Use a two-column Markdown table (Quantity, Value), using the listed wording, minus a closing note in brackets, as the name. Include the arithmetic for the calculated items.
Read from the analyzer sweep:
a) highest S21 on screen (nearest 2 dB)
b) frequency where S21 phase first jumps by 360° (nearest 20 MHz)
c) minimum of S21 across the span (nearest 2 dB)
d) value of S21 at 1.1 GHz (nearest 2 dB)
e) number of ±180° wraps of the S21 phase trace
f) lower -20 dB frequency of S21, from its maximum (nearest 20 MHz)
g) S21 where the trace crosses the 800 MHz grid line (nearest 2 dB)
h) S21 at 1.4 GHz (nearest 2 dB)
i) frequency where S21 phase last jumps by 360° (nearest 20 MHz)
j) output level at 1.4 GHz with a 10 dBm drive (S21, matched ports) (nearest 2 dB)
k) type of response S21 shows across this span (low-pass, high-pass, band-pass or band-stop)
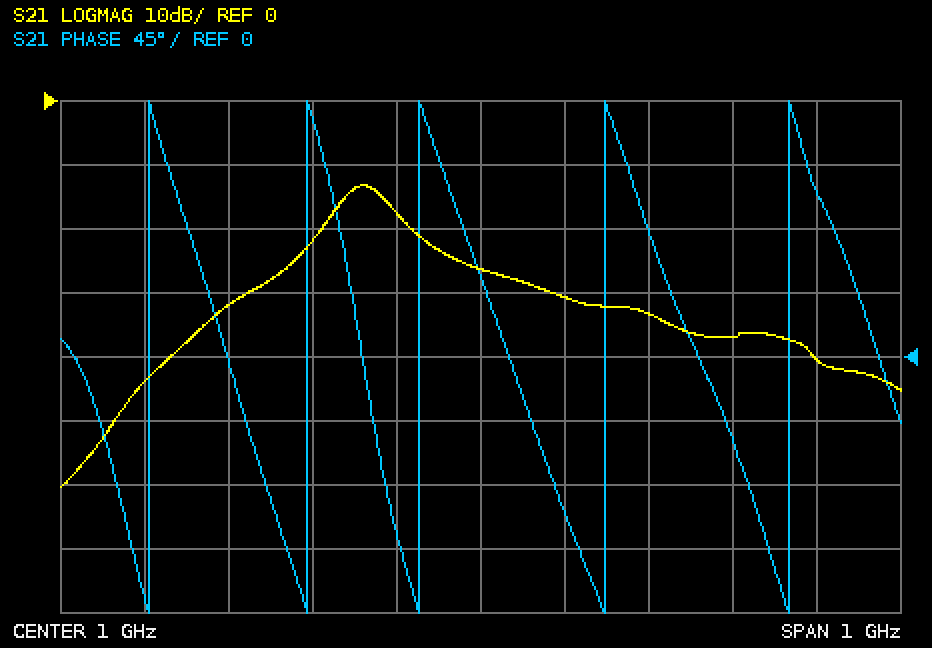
| Quantity | Value |
|---|---|
| highest S21 on screen | -14 dB |
| frequency where S21 phase first jumps by 360° | 600 MHz |
| minimum of S21 across the span | -60 dB |
| value of S21 at 1.1 GHz | -30 dB |
| number of ±180° wraps of the S21 phase trace | 5 |
| lower -20 dB frequency of S21, from its maximum | 680 MHz |
| S21 where the trace crosses the 800 MHz grid line | -22 dB |
| S21 at 1.4 GHz | -40 dB |
| frequency where S21 phase last jumps by 360° | 1.36 GHz |
| output level at 1.4 GHz with a 10 dBm drive (S21, matched ports) | 10 dBm + (-40 dB) = -30 dBm |
| type of response S21 shows across this span | band-pass |
